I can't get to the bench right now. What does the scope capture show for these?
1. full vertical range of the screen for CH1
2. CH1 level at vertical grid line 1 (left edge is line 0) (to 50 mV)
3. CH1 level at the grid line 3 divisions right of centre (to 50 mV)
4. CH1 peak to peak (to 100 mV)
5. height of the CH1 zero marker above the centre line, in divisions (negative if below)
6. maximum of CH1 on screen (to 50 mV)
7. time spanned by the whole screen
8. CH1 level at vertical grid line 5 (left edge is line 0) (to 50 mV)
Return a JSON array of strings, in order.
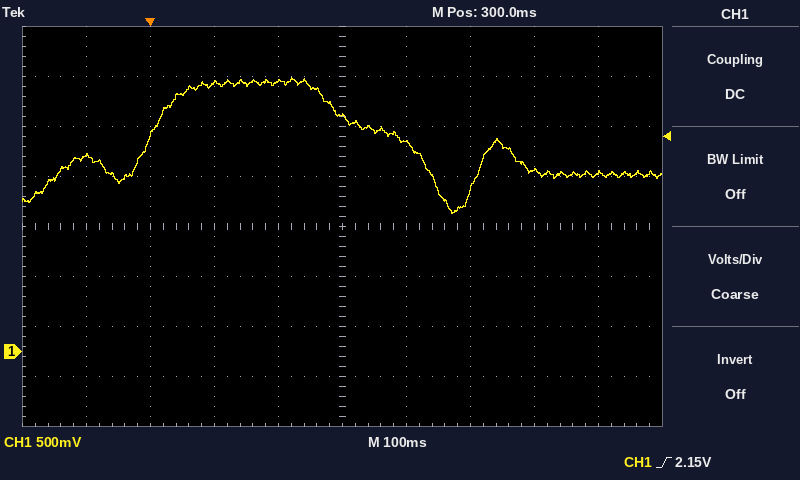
["4 V", "1.95 V", "1.80 V", "1.40 V", "-2.5 div", "2.75 V", "1 s", "2.35 V"]
